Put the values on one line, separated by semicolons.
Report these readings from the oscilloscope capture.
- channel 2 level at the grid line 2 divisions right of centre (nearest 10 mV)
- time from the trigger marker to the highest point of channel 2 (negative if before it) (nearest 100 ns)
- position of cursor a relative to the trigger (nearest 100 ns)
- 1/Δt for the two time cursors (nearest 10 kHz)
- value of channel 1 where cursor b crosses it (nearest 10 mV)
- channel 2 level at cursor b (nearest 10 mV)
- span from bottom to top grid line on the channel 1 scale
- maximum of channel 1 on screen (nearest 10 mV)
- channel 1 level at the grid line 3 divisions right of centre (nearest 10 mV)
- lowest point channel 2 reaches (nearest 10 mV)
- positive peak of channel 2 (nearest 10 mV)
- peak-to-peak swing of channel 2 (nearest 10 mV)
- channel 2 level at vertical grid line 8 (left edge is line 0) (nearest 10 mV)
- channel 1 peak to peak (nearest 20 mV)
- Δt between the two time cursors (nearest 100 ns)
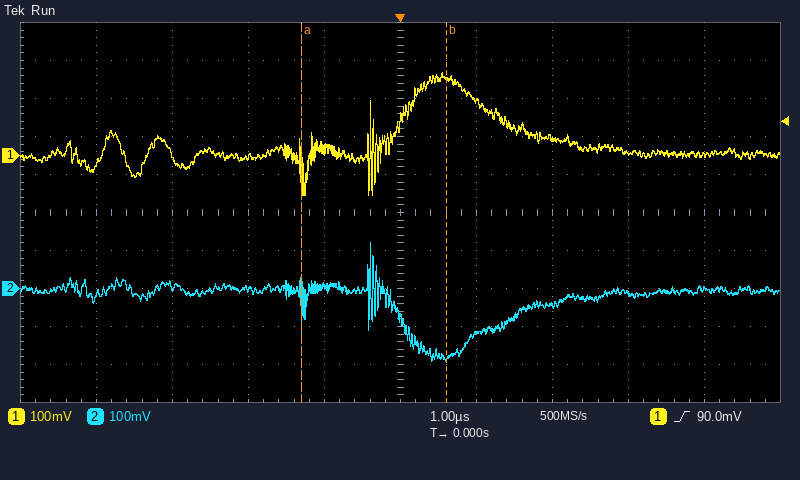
-40 mV; -400 ns; -1.3 µs; 530 kHz; 200 mV; -180 mV; 1 V; 220 mV; 10 mV; -190 mV; 120 mV; 310 mV; -10 mV; 320 mV; 1.9 µs
